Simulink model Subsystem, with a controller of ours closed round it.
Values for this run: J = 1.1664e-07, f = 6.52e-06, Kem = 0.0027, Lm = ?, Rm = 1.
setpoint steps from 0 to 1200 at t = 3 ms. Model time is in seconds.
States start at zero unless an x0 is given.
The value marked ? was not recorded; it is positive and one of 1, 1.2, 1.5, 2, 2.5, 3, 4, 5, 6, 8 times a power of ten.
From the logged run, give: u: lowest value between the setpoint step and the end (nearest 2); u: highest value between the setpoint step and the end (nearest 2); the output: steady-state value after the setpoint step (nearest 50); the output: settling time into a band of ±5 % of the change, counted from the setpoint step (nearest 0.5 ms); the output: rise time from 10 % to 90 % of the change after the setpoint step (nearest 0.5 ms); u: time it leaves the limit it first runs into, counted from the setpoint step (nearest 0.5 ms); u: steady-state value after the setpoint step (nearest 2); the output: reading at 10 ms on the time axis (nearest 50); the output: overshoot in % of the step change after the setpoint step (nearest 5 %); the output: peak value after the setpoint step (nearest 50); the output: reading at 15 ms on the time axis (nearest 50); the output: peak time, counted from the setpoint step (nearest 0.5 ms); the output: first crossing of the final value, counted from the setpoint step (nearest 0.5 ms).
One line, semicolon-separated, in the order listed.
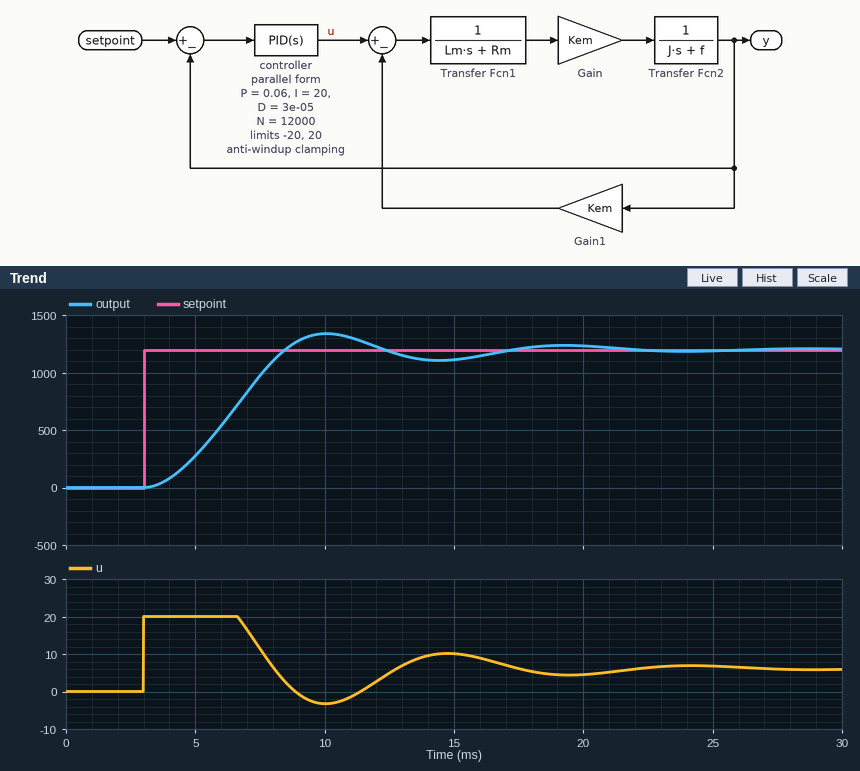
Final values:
-4; 20; 1200; 13.0 ms; 3.5 ms; 3.5 ms; 6; 1350; 10 %; 1350; 1100; 7.0 ms; 5.5 ms
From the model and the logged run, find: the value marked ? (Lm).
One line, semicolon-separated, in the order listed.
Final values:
0.0025
